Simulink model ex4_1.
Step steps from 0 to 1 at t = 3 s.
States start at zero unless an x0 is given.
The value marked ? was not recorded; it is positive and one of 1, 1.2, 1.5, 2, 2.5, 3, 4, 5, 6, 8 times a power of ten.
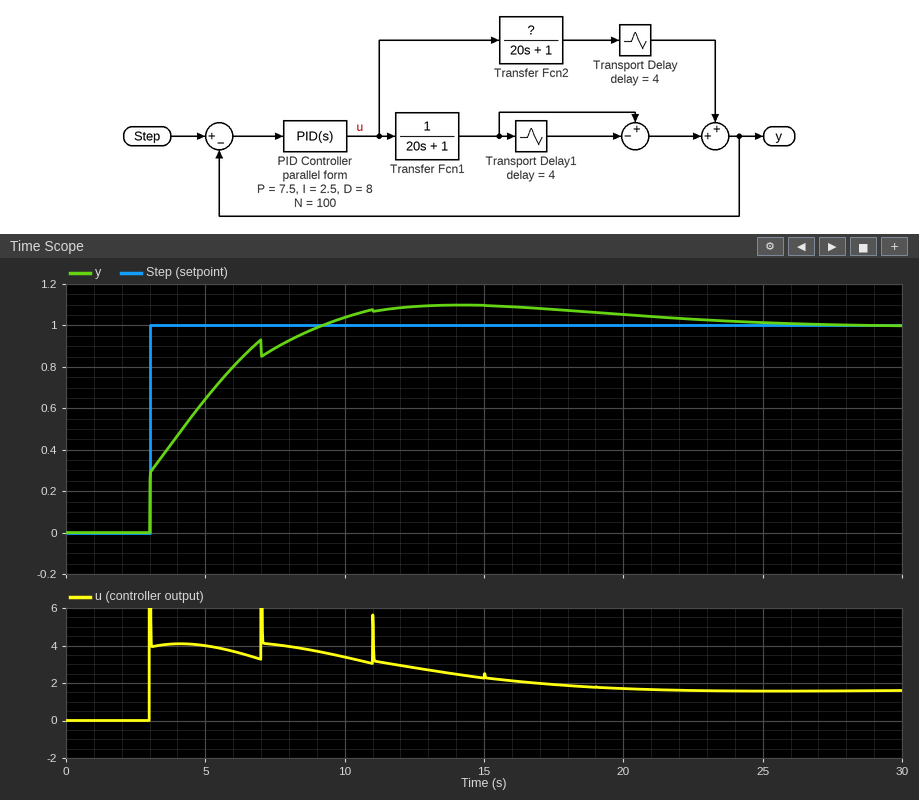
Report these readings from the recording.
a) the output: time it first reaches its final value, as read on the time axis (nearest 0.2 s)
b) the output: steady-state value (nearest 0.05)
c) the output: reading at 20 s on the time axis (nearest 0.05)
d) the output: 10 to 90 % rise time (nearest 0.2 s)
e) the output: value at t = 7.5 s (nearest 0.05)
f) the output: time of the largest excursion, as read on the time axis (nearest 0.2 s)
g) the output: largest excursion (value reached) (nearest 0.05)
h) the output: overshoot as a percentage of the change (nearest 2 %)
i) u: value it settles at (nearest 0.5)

9.2 s
1.00
1.05
3.8 s
0.90
14.2 s
1.10
10 %
1.5
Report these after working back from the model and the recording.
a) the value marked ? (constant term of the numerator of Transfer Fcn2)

0.6
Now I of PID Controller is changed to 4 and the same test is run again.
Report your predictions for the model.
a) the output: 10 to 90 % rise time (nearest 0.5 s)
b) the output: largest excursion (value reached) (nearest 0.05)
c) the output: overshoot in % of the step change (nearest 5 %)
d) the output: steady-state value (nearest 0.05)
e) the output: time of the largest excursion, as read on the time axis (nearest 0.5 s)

3.0 s
1.15
15 %
1.00
11.0 s
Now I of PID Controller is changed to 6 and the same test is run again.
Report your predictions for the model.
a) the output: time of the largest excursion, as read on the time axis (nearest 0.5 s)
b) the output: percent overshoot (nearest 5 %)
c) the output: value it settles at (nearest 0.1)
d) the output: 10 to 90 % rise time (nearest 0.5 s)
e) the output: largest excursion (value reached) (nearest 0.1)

9.0 s
15 %
1.0
2.5 s
1.2
